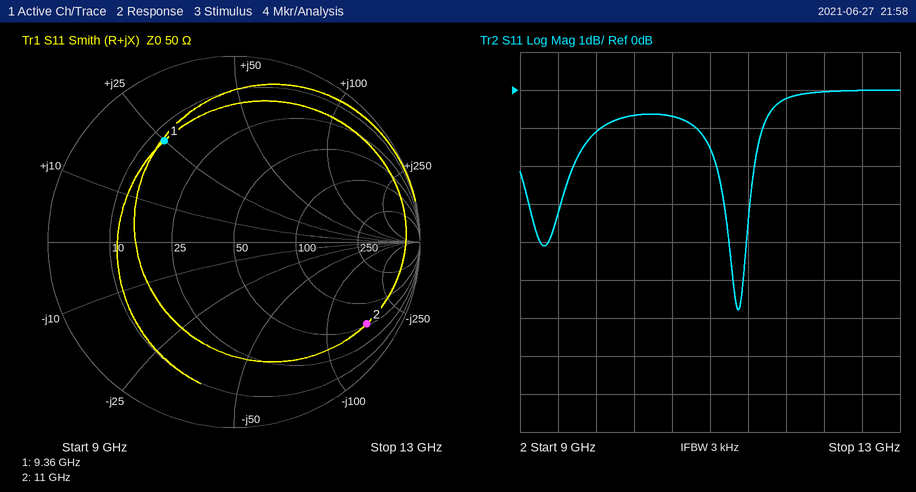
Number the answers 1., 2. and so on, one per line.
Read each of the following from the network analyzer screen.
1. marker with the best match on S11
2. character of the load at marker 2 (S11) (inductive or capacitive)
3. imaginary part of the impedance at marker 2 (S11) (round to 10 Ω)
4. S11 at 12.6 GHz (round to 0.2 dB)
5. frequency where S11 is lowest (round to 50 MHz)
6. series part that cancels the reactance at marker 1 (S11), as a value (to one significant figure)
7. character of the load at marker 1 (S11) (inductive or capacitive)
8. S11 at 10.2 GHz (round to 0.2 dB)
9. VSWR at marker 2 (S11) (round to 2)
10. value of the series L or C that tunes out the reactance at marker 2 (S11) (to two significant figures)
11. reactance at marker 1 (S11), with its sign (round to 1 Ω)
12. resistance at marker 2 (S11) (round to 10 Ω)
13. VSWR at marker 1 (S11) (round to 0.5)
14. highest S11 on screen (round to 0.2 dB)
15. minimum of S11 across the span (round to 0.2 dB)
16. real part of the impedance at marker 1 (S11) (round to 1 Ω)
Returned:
1. marker 1
2. capacitive
3. -160 Ω
4. 0.0 dB
5. 11.30 GHz
6. 700 fF
7. inductive
8. -0.6 dB
9. 12
10. 2.3 nH
11. +25 Ω
12. 50 Ω
13. 5.0
14. 0.0 dB
15. -5.8 dB
16. 13 Ω
